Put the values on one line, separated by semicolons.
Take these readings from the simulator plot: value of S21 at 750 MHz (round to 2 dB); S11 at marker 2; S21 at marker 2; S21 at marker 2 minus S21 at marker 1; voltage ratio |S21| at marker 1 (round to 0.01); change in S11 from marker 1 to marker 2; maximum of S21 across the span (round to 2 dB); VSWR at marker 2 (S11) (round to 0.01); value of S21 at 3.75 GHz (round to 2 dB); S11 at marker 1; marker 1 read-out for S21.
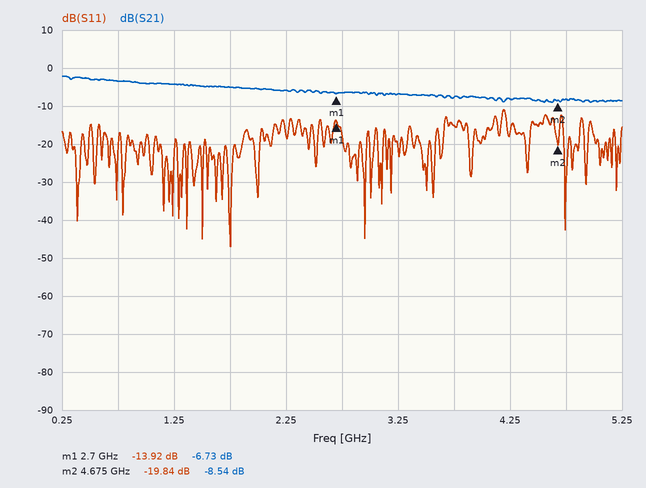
-4 dB; -19.84 dB; -8.54 dB; -1.81 dB; 0.46; -5.92 dB; -2 dB; 1.23; -8 dB; -13.92 dB; -6.73 dB
